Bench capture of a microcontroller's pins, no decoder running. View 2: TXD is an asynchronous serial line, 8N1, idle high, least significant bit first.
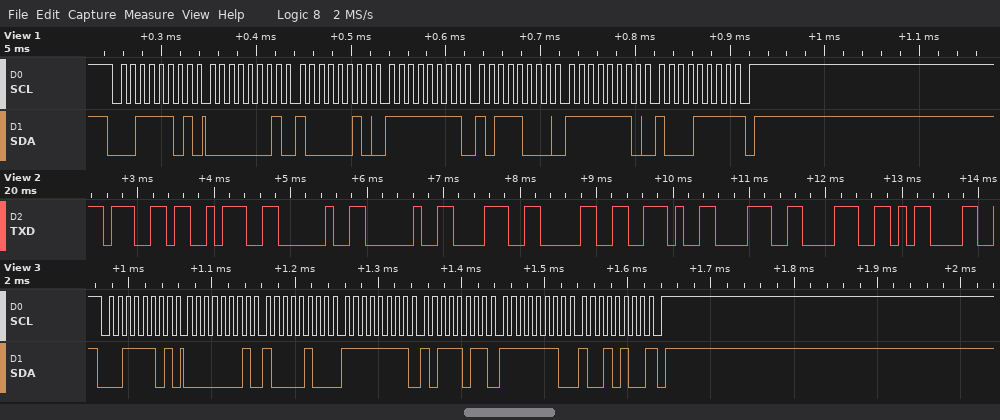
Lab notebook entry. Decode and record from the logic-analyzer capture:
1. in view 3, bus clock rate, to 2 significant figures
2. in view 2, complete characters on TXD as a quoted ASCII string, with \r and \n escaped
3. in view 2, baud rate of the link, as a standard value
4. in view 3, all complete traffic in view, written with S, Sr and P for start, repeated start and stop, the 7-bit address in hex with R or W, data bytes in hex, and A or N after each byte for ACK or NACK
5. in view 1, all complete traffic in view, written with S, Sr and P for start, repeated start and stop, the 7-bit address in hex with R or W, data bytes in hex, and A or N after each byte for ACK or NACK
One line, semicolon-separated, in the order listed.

100 kHz; "g:  80.88\r"; 9600 baud; S 1ER A 01 A 84 A FF A BB A FE A 94 N P; S 1ER A 01 A 82 A FF A B8 A FE A 8F N P
